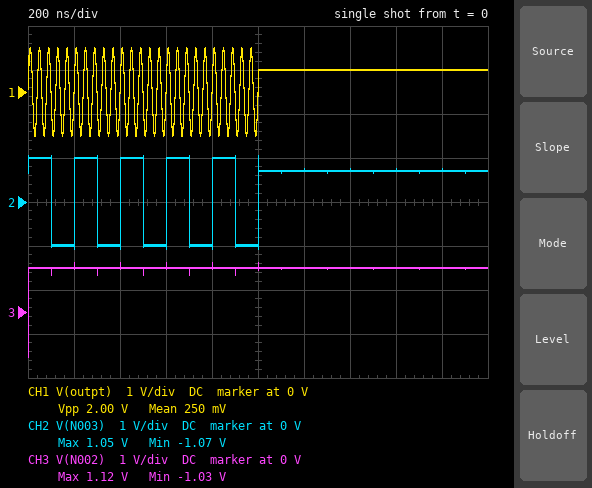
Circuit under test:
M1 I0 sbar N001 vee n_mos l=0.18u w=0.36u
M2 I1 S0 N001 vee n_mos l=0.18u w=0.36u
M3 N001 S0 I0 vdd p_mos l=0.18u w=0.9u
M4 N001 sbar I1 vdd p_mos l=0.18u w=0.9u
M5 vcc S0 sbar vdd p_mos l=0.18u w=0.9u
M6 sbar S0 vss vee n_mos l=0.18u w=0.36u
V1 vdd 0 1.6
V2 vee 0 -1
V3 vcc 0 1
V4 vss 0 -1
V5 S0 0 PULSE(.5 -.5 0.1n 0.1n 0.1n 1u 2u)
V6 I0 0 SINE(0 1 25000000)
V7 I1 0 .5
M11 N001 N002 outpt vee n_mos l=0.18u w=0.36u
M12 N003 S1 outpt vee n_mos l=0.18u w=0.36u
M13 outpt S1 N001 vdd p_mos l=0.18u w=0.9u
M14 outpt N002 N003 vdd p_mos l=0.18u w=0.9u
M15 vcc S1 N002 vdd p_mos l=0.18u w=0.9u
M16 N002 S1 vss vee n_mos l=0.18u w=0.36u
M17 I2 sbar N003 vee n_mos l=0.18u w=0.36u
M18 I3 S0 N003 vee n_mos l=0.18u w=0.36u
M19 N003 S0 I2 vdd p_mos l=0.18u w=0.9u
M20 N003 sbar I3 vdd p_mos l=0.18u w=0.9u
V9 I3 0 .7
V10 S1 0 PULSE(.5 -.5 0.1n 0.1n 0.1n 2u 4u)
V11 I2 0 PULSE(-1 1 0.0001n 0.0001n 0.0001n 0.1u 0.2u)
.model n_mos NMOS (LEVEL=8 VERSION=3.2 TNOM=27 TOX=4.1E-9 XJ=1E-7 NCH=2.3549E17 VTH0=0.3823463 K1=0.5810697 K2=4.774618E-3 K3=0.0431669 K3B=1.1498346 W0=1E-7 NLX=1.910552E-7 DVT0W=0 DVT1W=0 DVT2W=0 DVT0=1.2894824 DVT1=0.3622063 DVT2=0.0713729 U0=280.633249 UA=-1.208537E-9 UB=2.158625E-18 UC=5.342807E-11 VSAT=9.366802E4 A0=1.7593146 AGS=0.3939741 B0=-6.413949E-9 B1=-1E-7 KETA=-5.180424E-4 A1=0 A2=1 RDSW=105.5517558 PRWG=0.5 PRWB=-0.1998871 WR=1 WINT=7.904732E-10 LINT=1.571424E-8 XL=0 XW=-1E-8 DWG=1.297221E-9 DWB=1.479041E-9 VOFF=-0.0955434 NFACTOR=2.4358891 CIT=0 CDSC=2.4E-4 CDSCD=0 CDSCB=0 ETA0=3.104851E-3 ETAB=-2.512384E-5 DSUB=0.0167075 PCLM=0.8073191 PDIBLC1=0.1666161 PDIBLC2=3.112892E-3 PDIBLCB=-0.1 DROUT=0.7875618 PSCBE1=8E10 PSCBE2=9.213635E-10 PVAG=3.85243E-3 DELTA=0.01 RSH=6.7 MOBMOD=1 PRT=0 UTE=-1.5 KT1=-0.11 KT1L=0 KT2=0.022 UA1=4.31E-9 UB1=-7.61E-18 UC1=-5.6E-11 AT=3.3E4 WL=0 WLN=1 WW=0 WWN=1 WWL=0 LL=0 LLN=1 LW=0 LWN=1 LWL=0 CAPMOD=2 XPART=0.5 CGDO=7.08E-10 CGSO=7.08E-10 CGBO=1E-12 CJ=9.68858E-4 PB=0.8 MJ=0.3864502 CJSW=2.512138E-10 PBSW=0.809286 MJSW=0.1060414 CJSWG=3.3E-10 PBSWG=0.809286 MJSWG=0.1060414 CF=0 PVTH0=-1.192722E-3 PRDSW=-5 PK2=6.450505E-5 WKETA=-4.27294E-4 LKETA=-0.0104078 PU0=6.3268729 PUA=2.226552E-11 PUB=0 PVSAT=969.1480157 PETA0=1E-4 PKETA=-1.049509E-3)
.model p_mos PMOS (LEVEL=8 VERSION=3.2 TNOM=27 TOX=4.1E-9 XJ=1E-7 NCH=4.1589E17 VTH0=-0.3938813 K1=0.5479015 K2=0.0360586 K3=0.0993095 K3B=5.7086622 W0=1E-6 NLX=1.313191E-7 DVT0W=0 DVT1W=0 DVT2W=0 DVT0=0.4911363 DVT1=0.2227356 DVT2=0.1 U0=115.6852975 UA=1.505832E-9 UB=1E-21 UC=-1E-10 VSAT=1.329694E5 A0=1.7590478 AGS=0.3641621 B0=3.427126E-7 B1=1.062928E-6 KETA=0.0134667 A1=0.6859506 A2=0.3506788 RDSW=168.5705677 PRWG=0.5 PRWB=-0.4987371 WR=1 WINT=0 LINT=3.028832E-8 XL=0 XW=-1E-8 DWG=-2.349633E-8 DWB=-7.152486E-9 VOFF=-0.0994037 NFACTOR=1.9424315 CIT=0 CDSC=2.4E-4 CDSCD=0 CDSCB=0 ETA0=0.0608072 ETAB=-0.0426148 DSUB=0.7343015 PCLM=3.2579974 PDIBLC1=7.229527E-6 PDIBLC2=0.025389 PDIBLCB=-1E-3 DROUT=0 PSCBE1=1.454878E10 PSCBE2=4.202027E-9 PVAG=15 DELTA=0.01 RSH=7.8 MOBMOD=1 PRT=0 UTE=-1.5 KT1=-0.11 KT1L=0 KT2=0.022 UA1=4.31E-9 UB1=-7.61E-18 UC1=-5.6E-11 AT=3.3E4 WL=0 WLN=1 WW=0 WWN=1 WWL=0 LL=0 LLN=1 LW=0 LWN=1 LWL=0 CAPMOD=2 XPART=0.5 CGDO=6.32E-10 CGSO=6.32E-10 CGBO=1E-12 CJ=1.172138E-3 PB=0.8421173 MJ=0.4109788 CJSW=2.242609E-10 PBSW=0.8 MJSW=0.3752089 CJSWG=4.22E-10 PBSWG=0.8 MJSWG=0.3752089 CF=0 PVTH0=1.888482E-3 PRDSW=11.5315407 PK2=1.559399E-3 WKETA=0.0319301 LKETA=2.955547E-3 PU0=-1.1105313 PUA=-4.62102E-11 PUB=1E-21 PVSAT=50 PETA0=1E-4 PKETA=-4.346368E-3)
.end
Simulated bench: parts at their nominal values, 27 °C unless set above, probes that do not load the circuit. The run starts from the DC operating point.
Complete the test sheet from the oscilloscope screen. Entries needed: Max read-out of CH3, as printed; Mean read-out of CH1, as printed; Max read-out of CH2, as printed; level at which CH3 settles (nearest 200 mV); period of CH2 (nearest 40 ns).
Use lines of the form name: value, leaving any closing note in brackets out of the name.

Max read-out of CH3, as printed: 1.12 V
Mean read-out of CH1, as printed: 250 mV
Max read-out of CH2, as printed: 1.05 V
level at which CH3 settles: 1.0 V
period of CH2: 200 ns
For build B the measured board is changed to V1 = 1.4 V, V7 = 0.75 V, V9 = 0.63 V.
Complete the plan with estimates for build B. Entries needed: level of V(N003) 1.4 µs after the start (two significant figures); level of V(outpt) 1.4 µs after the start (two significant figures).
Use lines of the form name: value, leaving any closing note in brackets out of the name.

level of V(N003) 1.4 µs after the start: 630 mV
level of V(outpt) 1.4 µs after the start: 750 mV
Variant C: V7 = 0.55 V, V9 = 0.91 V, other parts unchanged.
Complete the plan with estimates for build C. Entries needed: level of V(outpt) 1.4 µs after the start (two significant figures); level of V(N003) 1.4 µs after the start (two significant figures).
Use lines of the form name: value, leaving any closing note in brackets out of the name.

level of V(outpt) 1.4 µs after the start: 550 mV
level of V(N003) 1.4 µs after the start: 910 mV
